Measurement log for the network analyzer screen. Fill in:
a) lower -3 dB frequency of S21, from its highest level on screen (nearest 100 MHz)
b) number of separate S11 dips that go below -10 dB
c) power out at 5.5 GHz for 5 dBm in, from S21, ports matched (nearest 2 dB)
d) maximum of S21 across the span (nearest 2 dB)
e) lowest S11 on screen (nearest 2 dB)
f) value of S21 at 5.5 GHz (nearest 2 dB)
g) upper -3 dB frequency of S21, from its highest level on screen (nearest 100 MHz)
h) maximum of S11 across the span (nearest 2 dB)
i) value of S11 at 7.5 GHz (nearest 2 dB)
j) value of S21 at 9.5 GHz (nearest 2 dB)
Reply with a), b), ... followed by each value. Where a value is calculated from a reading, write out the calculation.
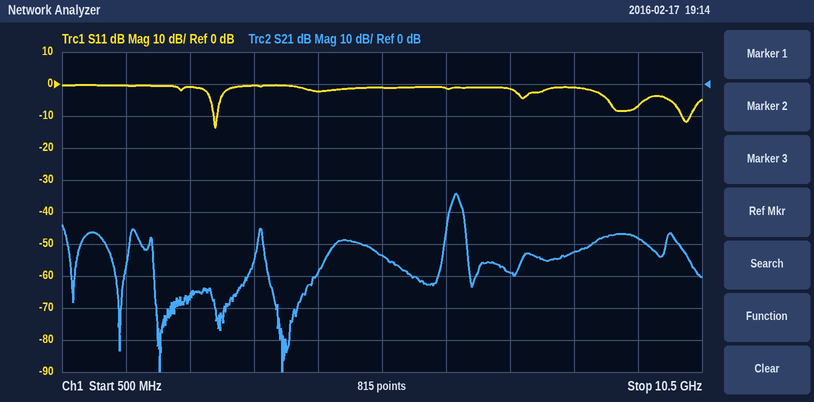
a) 6.6 GHz
b) 2
c) 5 dBm + (-54 dB) = -48 dBm
d) -34 dB
e) -14 dB
f) -54 dB
g) 6.7 GHz
h) 0 dB
i) -2 dB
j) -48 dB
